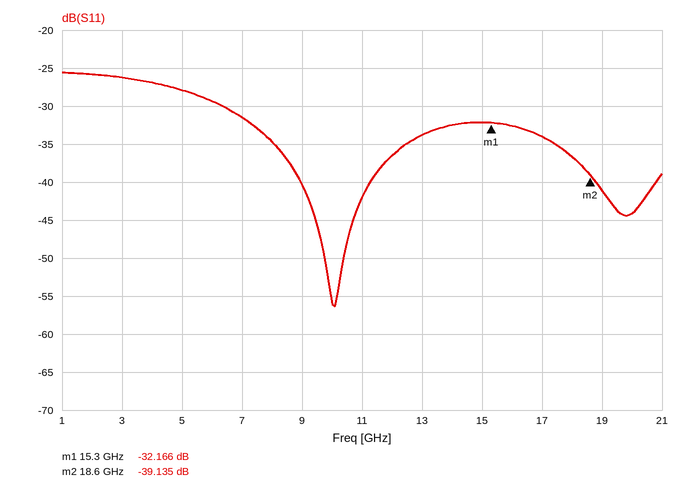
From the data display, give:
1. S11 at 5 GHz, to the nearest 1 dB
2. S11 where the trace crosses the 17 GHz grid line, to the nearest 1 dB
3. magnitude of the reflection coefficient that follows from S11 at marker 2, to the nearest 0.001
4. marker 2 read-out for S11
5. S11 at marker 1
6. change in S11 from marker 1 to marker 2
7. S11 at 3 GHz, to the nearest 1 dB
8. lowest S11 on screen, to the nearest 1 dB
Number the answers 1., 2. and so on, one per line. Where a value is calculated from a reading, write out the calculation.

1. -28 dB
2. -34 dB
3. 10^(-39.135/20) ≈ 0.011
4. -39.135 dB
5. -32.166 dB
6. -39.135 − (-32.166) = -6.969 dB
7. -26 dB
8. -56 dB
